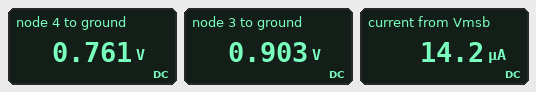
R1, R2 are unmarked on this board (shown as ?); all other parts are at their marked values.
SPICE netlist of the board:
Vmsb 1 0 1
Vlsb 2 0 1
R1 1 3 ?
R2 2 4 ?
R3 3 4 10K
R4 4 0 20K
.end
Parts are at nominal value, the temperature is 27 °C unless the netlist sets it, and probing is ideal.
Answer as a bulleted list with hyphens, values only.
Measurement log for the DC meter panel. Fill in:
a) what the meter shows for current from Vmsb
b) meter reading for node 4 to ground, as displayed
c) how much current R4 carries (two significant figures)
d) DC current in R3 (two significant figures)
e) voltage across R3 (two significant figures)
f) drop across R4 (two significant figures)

- 14.2 µA
- 0.761 V
- 38 µA
- 14 µA
- 140 mV
- 760 mV
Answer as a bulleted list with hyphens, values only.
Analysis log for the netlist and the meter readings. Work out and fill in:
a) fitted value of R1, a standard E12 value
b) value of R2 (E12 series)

- 6.8 kΩ
- 10 kΩ
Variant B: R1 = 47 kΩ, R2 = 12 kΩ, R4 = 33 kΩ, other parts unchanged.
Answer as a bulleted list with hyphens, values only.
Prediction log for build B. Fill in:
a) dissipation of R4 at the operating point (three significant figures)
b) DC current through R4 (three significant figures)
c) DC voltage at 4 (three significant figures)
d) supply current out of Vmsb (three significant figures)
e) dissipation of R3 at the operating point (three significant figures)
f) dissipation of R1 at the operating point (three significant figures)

- 17.9 µW
- 23.3 µA
- 769 mV
- 4.05 µA
- 164 nW
- 772 nW
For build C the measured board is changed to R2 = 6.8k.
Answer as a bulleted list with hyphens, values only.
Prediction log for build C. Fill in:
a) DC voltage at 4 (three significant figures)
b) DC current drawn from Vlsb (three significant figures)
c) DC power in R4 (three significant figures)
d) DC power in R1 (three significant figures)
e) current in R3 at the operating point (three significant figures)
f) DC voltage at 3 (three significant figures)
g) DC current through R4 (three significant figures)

- 805 mV
- 28.7 µA
- 32.4 µW
- 915 nW
- 11.6 µA
- 921 mV
- 40.3 µA
